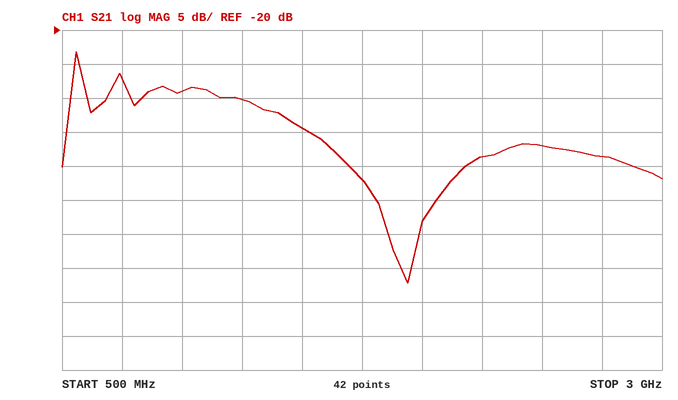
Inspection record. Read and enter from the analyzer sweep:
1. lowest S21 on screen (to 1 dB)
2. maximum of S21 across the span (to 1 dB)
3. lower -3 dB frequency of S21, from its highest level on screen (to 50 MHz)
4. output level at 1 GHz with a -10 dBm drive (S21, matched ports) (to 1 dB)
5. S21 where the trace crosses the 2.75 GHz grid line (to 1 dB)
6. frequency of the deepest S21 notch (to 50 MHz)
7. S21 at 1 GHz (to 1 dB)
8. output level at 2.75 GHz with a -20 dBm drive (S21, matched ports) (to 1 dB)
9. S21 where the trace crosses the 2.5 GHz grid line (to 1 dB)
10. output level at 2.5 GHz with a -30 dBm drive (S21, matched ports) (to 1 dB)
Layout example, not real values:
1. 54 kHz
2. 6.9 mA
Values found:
1. -57 dB
2. -23 dB
3. 550 MHz
4. -39 dBm
5. -39 dB
6. 1.95 GHz
7. -29 dB
8. -59 dBm
9. -37 dB
10. -67 dBm
